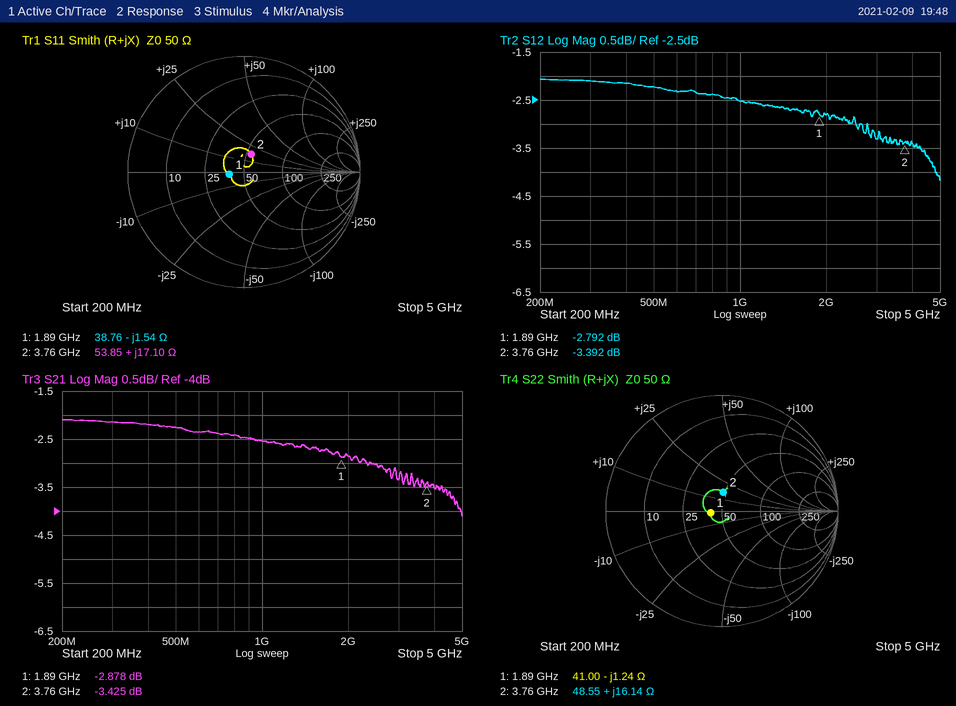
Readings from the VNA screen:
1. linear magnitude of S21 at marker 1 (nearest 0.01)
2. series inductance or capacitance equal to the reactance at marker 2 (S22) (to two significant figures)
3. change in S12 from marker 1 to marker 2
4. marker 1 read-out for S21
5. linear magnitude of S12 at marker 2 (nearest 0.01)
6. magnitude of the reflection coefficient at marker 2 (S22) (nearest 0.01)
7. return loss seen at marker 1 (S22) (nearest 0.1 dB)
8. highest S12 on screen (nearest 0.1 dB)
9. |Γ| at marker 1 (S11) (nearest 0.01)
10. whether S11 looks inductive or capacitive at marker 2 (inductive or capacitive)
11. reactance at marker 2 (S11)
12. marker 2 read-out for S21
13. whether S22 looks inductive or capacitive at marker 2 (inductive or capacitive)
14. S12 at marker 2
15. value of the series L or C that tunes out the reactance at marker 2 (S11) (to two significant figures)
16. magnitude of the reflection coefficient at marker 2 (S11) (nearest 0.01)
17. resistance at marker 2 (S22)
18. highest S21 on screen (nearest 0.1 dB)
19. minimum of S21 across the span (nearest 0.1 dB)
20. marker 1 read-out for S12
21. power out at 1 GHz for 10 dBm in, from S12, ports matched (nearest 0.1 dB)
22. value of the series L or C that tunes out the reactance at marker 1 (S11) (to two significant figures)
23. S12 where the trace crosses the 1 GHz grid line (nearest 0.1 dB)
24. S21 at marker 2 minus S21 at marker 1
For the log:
0.72
680 pH
-0.600 dB
-2.878 dB
0.68
0.16
20.0 dB
-2.1 dB
0.13
inductive
+17.10 Ω
-3.425 dB
inductive
-3.392 dB
2.5 pF
0.17
48.55 Ω
-2.1 dB
-4.1 dB
-2.792 dB
7.5 dBm
130 pH
-2.5 dB
-0.547 dB
